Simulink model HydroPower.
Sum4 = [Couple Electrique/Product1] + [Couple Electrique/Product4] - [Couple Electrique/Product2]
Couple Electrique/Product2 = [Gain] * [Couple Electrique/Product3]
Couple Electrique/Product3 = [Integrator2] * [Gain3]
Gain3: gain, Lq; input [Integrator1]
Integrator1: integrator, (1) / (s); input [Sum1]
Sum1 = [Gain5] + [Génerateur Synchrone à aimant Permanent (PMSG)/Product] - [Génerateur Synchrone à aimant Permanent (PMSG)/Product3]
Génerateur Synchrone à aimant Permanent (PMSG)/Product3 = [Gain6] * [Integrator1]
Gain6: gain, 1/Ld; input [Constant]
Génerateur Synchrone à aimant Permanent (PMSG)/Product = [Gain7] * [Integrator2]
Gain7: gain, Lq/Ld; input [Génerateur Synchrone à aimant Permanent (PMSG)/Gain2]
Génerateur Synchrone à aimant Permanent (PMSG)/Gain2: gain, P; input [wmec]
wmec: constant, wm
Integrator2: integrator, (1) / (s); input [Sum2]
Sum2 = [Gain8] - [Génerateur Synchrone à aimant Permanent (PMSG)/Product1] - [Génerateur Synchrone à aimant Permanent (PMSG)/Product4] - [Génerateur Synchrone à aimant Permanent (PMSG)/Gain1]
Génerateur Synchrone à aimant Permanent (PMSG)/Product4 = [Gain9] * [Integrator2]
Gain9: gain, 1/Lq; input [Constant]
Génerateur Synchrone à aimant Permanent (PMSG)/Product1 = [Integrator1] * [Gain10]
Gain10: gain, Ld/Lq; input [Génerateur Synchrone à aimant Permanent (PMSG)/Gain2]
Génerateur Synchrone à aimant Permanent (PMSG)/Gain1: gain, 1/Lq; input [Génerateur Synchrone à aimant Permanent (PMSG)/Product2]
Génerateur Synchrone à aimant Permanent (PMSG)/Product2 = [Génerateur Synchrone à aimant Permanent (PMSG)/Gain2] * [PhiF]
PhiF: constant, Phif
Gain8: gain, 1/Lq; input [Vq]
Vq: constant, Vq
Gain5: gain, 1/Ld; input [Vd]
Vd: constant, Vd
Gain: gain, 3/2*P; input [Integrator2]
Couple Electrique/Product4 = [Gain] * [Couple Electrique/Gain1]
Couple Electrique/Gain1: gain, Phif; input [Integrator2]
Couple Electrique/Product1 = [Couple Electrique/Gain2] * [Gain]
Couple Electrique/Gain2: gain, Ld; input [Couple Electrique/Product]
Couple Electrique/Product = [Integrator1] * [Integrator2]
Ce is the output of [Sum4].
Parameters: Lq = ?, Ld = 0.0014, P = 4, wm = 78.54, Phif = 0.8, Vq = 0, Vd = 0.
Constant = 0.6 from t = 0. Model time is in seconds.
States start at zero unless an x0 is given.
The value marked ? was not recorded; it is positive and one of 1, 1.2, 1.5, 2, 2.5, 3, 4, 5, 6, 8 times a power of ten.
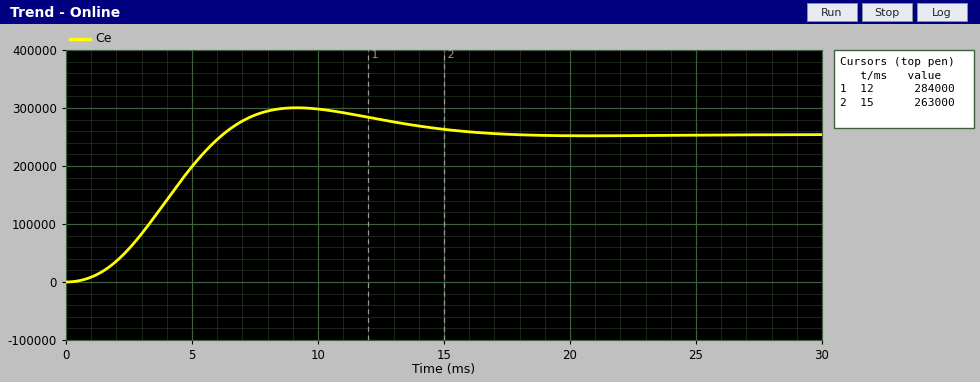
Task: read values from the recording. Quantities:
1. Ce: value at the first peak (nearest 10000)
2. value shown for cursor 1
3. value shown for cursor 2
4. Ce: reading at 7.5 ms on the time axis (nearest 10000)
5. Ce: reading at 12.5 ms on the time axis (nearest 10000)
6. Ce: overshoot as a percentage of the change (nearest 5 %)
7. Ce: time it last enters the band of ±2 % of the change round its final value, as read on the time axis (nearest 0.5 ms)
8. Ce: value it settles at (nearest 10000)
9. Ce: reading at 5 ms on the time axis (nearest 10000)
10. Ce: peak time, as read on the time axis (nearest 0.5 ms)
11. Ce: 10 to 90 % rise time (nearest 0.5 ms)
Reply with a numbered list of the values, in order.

1. 300000
2. 284000
3. 263000
4. 290000
5. 280000
6. 20 %
7. 16.0 ms
8. 250000
9. 200000
10. 9.0 ms
11. 4.0 ms
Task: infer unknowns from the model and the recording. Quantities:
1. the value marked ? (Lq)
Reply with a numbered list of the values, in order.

1. 0.006
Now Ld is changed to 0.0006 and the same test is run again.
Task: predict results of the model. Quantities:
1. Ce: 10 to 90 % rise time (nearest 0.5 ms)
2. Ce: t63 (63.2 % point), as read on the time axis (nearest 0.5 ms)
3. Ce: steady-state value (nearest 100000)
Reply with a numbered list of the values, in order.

1. 12.0 ms
2. 9.0 ms
3. 1200000
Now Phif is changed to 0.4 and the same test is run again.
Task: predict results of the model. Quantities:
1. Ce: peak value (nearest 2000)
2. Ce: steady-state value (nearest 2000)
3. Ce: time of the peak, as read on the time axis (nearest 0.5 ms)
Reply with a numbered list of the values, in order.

1. 38000
2. 32000
3. 9.0 ms
